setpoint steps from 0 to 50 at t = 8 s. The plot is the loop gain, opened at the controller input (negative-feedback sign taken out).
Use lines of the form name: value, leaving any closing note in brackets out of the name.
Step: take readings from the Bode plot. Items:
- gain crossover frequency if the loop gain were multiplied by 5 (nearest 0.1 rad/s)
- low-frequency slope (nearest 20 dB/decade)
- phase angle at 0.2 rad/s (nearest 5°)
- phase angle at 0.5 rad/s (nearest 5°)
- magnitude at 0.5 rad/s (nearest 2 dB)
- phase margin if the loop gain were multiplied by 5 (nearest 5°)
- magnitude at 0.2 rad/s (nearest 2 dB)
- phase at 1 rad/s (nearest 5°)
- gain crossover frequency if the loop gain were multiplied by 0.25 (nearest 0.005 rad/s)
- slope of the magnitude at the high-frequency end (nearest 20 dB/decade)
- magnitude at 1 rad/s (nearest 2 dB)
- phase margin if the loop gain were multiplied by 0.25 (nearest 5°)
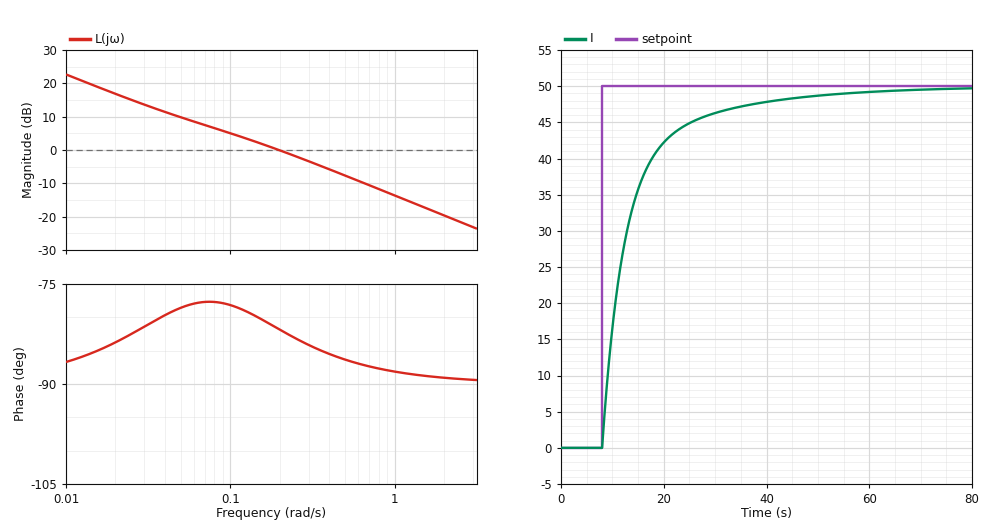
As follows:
gain crossover frequency if the loop gain were multiplied by 5: 1.0 rad/s
low-frequency slope: -20 dB/decade
phase angle at 0.2 rad/s: -80°
phase angle at 0.5 rad/s: -85°
magnitude at 0.5 rad/s: -8 dB
phase margin if the loop gain were multiplied by 5: 90°
magnitude at 0.2 rad/s: 0 dB
phase at 1 rad/s: -90°
gain crossover frequency if the loop gain were multiplied by 0.25: 0.035 rad/s
slope of the magnitude at the high-frequency end: -20 dB/decade
magnitude at 1 rad/s: -14 dB
phase margin if the loop gain were multiplied by 0.25: 100°
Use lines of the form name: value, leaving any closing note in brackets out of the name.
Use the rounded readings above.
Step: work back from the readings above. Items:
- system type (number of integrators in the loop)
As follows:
system type: 1
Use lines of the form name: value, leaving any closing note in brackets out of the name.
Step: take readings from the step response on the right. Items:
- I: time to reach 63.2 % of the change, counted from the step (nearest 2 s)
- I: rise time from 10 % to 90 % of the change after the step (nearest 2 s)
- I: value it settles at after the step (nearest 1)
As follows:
I: time to reach 63.2 % of the change, counted from the step: 6 s
I: rise time from 10 % to 90 % of the change after the step: 16 s
I: value it settles at after the step: 50
